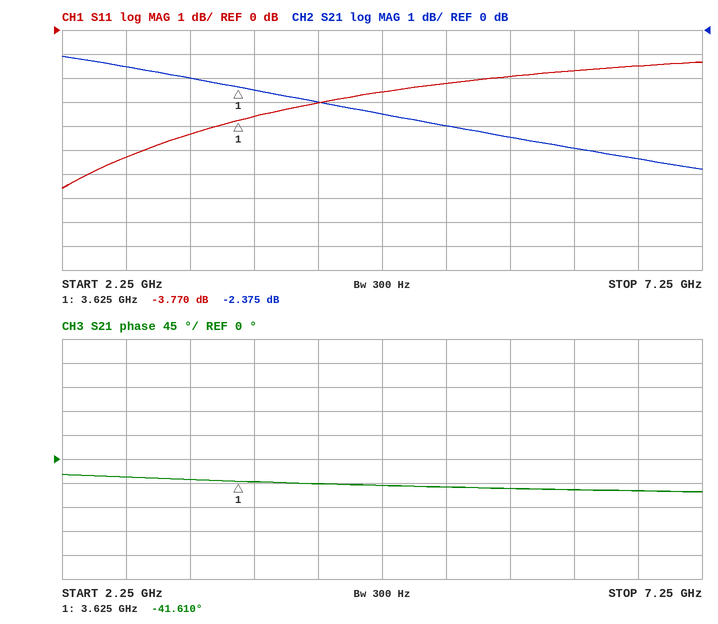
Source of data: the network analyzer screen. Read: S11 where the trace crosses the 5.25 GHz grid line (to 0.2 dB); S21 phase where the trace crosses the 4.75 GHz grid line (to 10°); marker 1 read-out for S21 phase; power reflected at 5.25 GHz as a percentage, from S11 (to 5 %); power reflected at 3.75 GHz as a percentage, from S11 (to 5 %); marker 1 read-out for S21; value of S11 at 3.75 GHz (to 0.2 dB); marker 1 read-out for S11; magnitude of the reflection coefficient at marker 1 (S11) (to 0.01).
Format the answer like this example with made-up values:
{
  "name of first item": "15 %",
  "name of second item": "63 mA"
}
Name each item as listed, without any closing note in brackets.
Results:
{
  "S11 where the trace crosses the 5.25 GHz grid line": "-2.2 dB",
  "S21 phase where the trace crosses the 4.75 GHz grid line": "-50°",
  "marker 1 read-out for S21 phase": "-41.610°",
  "power reflected at 5.25 GHz as a percentage, from S11": "60 %",
  "power reflected at 3.75 GHz as a percentage, from S11": "45 %",
  "marker 1 read-out for S21": "-2.375 dB",
  "value of S11 at 3.75 GHz": "-3.6 dB",
  "marker 1 read-out for S11": "-3.770 dB",
  "magnitude of the reflection coefficient at marker 1 (S11)": "0.65"
}
